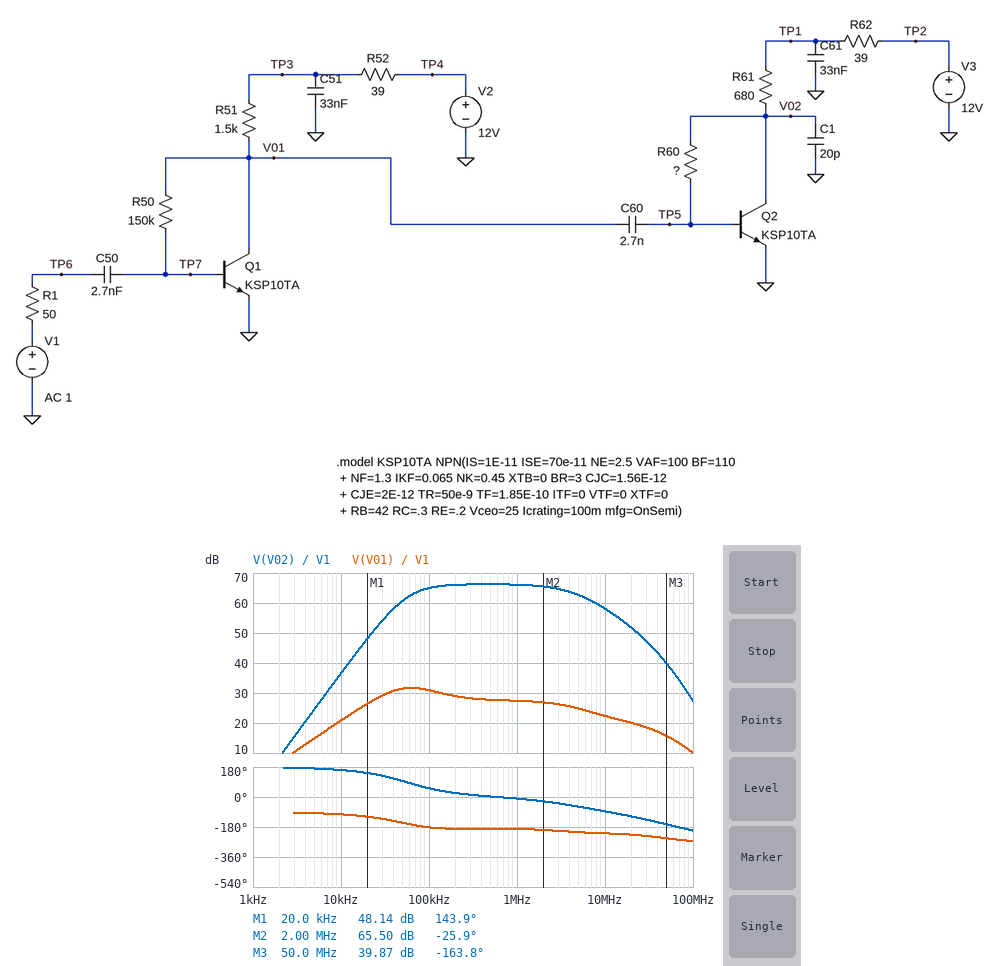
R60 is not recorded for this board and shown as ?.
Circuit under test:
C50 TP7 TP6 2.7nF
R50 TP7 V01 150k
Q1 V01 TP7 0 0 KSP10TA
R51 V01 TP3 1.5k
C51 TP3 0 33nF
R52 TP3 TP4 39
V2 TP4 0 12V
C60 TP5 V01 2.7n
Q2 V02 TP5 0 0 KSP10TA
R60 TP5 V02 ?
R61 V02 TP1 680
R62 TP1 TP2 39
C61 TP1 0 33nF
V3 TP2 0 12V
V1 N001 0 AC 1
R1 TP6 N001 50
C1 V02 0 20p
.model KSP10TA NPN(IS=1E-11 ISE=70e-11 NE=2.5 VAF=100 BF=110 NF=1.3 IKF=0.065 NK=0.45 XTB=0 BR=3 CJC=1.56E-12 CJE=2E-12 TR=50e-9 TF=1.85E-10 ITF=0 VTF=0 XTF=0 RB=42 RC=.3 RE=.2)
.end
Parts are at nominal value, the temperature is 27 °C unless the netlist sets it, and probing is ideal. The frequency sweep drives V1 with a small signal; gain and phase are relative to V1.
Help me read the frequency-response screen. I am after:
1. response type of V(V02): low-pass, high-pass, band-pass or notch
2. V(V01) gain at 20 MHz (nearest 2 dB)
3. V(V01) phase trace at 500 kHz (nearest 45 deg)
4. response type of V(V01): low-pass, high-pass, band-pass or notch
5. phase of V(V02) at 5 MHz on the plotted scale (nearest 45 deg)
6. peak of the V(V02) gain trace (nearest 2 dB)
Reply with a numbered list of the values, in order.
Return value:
1. band-pass
2. 20 dB
3. -180 deg
4. band-pass
5. -45 deg
6. 66 dB
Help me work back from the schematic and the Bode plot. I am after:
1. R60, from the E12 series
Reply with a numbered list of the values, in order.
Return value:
1. 100 kΩ
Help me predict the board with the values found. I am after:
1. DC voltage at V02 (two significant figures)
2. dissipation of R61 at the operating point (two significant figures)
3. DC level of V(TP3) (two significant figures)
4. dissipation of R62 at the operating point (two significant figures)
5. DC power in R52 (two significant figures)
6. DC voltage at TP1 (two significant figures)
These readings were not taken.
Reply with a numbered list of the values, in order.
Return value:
1. 8.0 V
2. 21 mW
3. 12 V
4. 1.2 mW
5. 360 µW
6. 12 V
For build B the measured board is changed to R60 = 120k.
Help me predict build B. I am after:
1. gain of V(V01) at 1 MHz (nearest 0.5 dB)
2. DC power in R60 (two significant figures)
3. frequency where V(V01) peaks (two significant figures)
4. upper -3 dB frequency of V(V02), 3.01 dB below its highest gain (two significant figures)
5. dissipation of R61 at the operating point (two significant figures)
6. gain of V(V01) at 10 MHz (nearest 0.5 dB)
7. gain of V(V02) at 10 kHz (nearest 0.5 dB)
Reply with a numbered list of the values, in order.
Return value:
1. 28.5 dB
2. 510 µW
3. 65 kHz
4. 4.3 MHz
5. 16 mW
6. 23.0 dB
7. 37.0 dB
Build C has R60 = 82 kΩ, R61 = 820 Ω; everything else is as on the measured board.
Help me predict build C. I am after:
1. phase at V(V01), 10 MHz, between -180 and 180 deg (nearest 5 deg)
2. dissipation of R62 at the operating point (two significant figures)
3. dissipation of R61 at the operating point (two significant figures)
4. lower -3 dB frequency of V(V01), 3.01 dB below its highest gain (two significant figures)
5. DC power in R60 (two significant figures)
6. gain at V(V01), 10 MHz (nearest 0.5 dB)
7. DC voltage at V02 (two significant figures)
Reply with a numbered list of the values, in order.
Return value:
1. 145 deg
2. 1.3 mW
3. 27 mW
4. 28 kHz
5. 490 µW
6. 21.5 dB
7. 7.0 V
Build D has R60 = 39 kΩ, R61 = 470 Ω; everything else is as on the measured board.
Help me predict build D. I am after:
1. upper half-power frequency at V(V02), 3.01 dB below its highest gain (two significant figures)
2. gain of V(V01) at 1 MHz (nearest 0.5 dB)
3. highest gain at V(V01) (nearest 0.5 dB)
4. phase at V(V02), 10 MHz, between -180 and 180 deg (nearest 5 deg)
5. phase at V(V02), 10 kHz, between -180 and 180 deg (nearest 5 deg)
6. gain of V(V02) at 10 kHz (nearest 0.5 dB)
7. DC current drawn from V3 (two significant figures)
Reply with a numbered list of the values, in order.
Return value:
1. 6.9 MHz
2. 22.0 dB
3. 32.5 dB
4. -75 deg
5. 165 deg
6. 31.0 dB
7. 11 mA
